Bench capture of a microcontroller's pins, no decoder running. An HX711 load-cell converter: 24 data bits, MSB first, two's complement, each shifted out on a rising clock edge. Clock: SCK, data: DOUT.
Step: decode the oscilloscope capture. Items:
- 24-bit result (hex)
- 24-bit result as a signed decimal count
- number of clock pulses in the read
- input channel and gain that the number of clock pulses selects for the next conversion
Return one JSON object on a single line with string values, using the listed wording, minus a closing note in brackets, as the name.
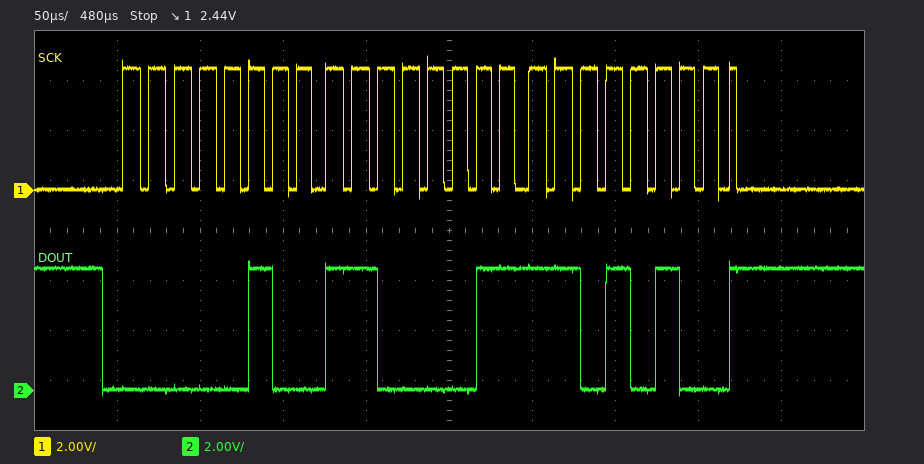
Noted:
{"24-bit result": "0x04C3D4", "24-bit result as a signed decimal count": "312276", "number of clock pulses in the read": "25", "input channel and gain that the number of clock pulses selects for the next conversion": "channel A, gain 128"}
